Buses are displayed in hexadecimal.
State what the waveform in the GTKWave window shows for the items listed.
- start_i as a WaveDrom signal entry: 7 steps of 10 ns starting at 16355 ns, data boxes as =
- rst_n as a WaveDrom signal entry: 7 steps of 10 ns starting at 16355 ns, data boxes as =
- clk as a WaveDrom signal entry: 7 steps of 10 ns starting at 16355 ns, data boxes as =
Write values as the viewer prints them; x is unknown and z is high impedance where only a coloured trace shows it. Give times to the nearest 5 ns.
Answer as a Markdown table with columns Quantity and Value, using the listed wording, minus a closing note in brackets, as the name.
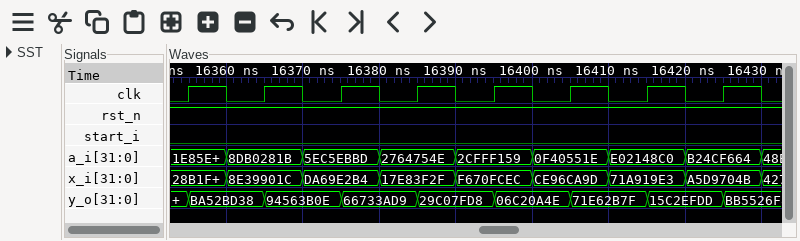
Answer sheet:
| Quantity | Value |
|---|---|
| start_i as a WaveDrom signal entry: 7 steps of 10 ns starting at 16355 ns, data boxes as = | {name: 'start_i', wave: '0......'} |
| rst_n as a WaveDrom signal entry: 7 steps of 10 ns starting at 16355 ns, data boxes as = | {name: 'rst_n', wave: '1......'} |
| clk as a WaveDrom signal entry: 7 steps of 10 ns starting at 16355 ns, data boxes as = | {name: 'clk', wave: 'p......'} |
